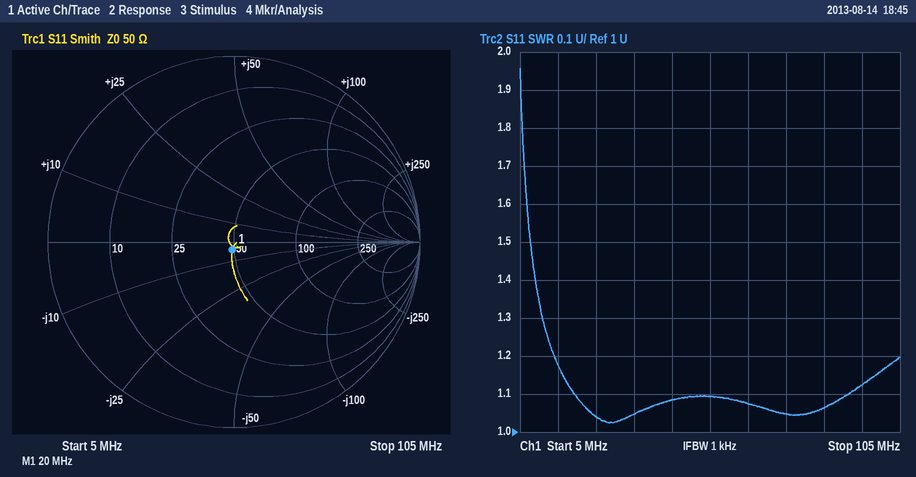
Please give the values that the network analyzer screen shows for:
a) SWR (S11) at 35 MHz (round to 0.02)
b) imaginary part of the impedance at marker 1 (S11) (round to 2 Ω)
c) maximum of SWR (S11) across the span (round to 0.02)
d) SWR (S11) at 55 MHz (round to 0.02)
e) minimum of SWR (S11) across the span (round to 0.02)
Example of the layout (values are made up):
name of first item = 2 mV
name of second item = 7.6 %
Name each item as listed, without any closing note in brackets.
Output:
SWR (S11) at 35 MHz = 1.04
imaginary part of the impedance at marker 1 (S11) = -4 Ω
maximum of SWR (S11) across the span = 1.96
SWR (S11) at 55 MHz = 1.10
minimum of SWR (S11) across the span = 1.02
